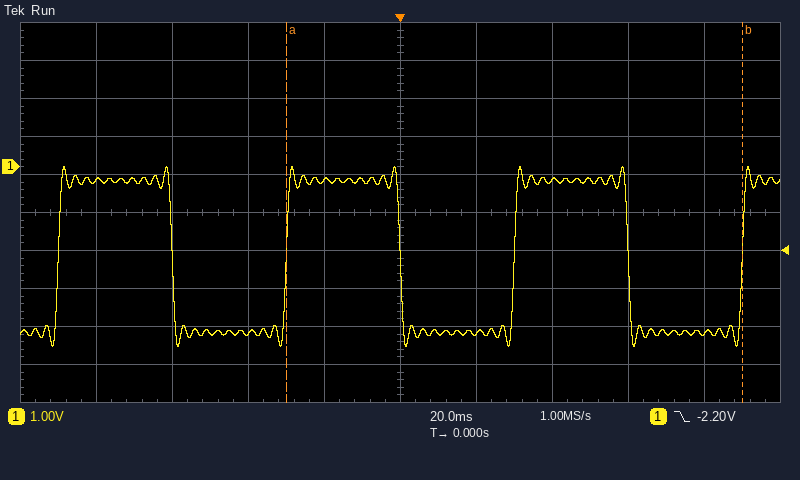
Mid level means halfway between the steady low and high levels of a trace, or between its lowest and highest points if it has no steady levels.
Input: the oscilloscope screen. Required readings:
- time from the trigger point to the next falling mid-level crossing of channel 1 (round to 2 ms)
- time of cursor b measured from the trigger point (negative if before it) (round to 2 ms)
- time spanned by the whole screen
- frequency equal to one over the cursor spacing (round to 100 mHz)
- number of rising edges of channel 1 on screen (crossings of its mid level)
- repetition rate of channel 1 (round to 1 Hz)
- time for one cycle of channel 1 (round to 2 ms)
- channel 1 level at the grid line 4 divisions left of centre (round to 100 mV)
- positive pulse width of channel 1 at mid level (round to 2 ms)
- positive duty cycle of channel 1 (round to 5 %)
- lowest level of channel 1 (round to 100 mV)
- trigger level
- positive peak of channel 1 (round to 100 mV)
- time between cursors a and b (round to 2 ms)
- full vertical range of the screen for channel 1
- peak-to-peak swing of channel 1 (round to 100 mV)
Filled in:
60 ms
+90 ms
200 ms
8.3 Hz
4
17 Hz
60 ms
-400 mV
30 ms
50 %
-4.7 V
-2.20 V
0.0 V
120 ms
10 V
4.7 V
